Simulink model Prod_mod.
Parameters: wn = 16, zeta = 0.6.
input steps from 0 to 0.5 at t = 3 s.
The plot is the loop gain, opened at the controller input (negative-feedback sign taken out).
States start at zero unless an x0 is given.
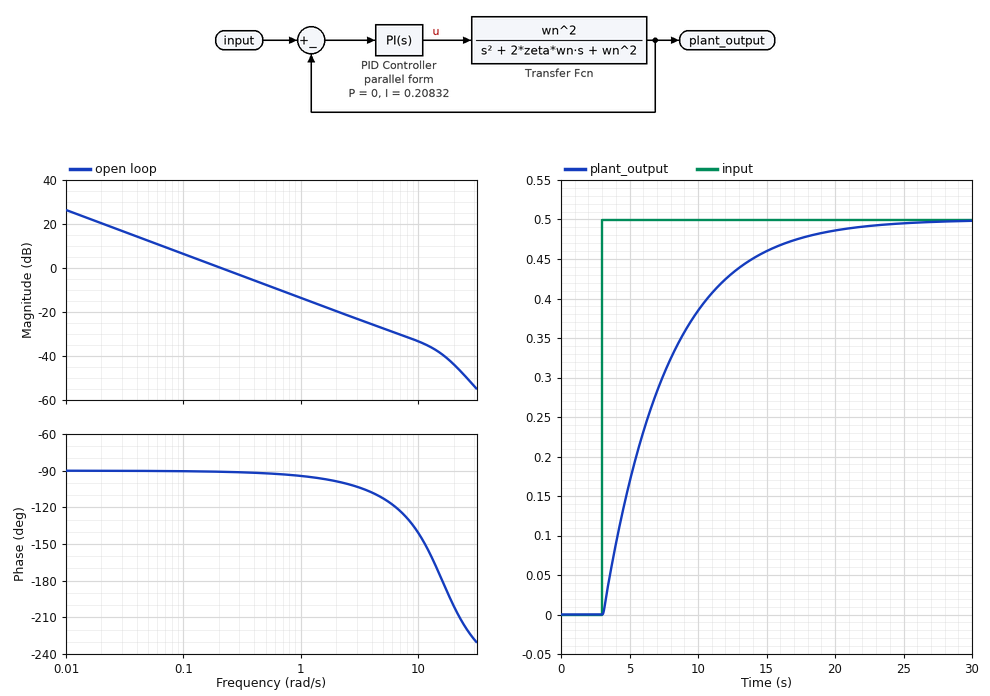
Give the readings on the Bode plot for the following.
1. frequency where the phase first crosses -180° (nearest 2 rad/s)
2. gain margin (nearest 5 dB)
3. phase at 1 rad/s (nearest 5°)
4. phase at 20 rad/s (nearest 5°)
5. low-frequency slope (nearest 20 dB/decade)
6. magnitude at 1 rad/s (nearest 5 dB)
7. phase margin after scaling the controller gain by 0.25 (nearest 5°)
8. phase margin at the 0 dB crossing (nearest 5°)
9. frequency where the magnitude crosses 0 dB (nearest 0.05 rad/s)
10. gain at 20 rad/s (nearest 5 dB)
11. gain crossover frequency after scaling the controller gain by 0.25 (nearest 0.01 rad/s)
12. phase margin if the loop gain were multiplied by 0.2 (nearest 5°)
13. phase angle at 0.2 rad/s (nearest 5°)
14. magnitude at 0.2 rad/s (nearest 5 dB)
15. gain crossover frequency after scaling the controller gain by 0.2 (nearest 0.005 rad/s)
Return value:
16 rad/s
40 dB
-95°
-200°
-20 dB/decade
-15 dB
90°
90°
0.20 rad/s
-45 dB
0.05 rad/s
90°
-90°
0 dB
0.040 rad/s
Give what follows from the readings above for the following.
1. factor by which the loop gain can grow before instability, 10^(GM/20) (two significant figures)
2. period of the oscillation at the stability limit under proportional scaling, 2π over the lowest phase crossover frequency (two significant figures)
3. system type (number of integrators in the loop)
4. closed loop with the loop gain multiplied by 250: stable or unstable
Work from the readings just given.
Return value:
100
0.39 s
1
unstable
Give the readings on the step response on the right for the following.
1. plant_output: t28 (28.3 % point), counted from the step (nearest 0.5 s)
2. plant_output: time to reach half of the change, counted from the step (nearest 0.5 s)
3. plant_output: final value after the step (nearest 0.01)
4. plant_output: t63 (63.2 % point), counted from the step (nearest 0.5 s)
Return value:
1.5 s
3.5 s
0.50
5.0 s
